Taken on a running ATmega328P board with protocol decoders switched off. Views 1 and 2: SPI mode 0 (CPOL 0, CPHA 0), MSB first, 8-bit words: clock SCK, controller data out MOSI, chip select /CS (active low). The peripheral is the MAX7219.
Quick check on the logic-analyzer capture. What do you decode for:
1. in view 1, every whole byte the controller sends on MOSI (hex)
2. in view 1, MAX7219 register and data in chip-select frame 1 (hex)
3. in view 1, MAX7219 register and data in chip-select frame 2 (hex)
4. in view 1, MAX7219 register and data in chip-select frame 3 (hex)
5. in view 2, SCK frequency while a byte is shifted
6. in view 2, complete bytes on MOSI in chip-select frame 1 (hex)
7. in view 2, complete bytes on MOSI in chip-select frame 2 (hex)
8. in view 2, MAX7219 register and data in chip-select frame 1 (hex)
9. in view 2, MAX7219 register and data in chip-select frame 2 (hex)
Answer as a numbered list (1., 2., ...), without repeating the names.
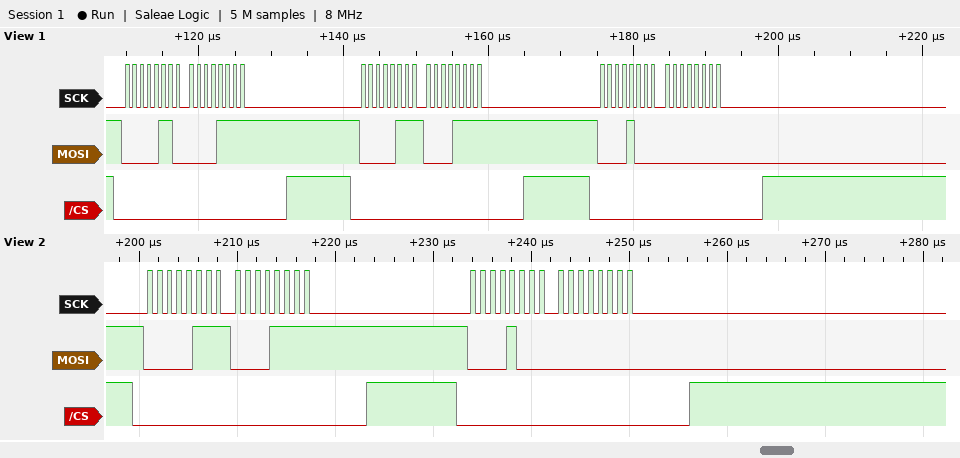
1. 06 0F 07 0F 08 00
2. register 0x6, data 0x0F
3. register 0x7, data 0x0F
4. register 0x8, data 0x00
5. 1 MHz
6. 07 0F
7. 08 00
8. register 0x7, data 0x0F
9. register 0x8, data 0x00
